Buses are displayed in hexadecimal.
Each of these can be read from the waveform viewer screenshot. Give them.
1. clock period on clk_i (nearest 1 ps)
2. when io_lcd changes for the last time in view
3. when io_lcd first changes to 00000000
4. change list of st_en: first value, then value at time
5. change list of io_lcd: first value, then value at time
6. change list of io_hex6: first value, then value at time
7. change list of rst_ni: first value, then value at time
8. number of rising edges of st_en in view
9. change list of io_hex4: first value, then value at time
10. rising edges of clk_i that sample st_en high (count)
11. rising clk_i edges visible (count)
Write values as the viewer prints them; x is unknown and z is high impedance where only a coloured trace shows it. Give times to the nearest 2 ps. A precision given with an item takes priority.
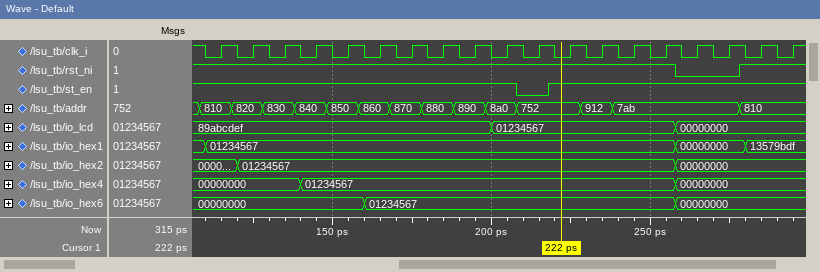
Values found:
10 ps
258 ps
258 ps
1, 0 at 208 ps, 1 at 218 ps
89abcdef, 01234567 at 200 ps, 00000000 at 258 ps
00000000, 01234567 at 160 ps, 00000000 at 258 ps
1, 0 at 258 ps, 1 at 278 ps
1
00000000, 01234567 at 140 ps, 00000000 at 258 ps
18
19
